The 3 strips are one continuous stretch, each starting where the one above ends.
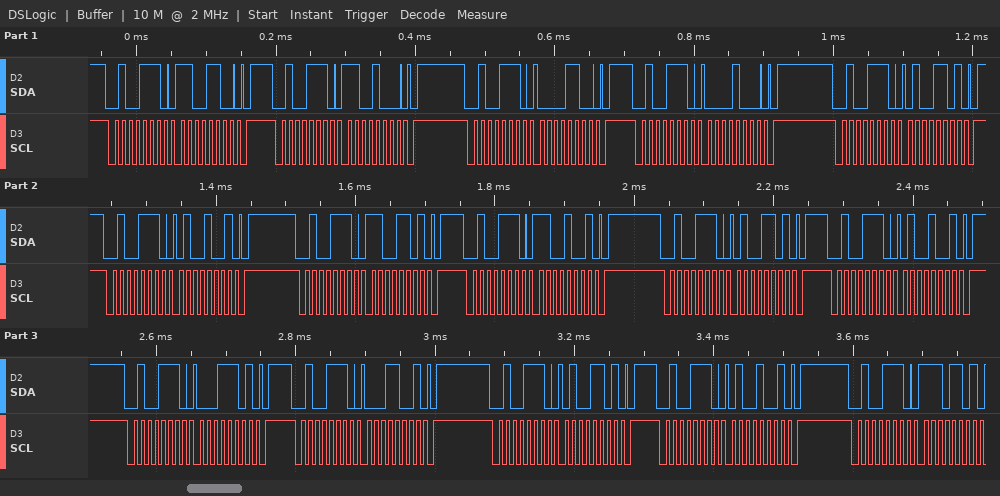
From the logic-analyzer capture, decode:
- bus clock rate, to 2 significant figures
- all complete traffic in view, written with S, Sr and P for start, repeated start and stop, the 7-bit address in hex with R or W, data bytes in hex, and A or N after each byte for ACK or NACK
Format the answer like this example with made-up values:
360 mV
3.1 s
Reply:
100 kHz
S 27W A CC A P S 27W A C8 A P S 27W A 0C A P S 27W A 08 A P S 27W A 4D A P S 27W A 49 A P S 27W A CD A P S 27W A C9 A P S 27W A 4D A P S 27W A 49 A P S 27W A 1D A P S 27W A 19 A P S 27W A 4D A P S 27W A 49 A P S 27W A ED A
